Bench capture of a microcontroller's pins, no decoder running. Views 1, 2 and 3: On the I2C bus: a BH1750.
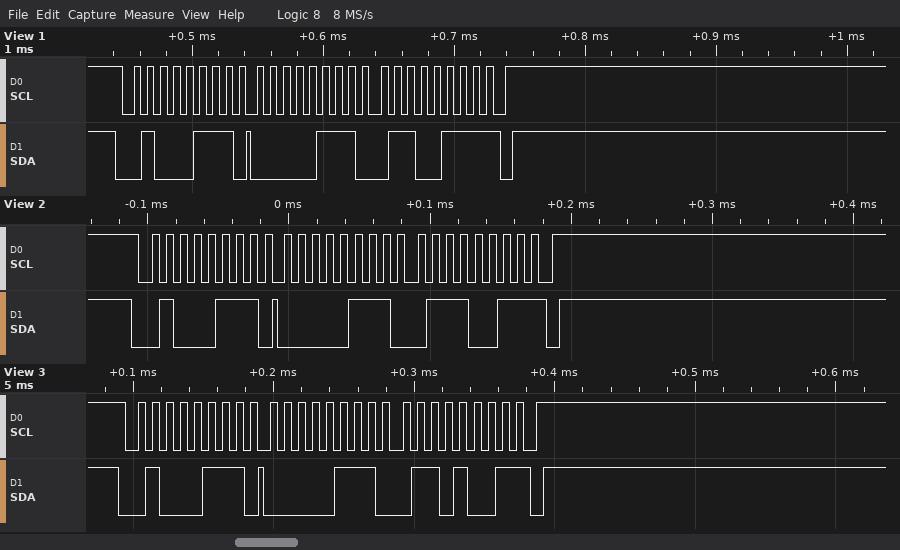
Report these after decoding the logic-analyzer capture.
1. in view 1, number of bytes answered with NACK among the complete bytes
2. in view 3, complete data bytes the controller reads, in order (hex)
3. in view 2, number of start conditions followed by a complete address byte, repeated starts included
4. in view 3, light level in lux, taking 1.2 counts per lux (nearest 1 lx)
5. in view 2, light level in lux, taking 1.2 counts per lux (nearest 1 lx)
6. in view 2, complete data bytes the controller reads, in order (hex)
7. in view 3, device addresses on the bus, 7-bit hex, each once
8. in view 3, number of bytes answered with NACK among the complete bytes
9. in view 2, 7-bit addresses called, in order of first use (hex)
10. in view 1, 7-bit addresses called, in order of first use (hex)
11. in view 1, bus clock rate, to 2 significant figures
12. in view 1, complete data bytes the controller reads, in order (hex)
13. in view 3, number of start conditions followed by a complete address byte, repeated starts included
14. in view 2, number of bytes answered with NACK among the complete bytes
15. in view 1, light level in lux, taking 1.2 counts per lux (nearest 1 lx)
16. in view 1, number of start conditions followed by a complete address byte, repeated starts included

1
07 69
1
1581 lx
1589 lx
07 73
0x23
1
0x23
0x23
100 kHz
07 67
1
1
1579 lx
1
